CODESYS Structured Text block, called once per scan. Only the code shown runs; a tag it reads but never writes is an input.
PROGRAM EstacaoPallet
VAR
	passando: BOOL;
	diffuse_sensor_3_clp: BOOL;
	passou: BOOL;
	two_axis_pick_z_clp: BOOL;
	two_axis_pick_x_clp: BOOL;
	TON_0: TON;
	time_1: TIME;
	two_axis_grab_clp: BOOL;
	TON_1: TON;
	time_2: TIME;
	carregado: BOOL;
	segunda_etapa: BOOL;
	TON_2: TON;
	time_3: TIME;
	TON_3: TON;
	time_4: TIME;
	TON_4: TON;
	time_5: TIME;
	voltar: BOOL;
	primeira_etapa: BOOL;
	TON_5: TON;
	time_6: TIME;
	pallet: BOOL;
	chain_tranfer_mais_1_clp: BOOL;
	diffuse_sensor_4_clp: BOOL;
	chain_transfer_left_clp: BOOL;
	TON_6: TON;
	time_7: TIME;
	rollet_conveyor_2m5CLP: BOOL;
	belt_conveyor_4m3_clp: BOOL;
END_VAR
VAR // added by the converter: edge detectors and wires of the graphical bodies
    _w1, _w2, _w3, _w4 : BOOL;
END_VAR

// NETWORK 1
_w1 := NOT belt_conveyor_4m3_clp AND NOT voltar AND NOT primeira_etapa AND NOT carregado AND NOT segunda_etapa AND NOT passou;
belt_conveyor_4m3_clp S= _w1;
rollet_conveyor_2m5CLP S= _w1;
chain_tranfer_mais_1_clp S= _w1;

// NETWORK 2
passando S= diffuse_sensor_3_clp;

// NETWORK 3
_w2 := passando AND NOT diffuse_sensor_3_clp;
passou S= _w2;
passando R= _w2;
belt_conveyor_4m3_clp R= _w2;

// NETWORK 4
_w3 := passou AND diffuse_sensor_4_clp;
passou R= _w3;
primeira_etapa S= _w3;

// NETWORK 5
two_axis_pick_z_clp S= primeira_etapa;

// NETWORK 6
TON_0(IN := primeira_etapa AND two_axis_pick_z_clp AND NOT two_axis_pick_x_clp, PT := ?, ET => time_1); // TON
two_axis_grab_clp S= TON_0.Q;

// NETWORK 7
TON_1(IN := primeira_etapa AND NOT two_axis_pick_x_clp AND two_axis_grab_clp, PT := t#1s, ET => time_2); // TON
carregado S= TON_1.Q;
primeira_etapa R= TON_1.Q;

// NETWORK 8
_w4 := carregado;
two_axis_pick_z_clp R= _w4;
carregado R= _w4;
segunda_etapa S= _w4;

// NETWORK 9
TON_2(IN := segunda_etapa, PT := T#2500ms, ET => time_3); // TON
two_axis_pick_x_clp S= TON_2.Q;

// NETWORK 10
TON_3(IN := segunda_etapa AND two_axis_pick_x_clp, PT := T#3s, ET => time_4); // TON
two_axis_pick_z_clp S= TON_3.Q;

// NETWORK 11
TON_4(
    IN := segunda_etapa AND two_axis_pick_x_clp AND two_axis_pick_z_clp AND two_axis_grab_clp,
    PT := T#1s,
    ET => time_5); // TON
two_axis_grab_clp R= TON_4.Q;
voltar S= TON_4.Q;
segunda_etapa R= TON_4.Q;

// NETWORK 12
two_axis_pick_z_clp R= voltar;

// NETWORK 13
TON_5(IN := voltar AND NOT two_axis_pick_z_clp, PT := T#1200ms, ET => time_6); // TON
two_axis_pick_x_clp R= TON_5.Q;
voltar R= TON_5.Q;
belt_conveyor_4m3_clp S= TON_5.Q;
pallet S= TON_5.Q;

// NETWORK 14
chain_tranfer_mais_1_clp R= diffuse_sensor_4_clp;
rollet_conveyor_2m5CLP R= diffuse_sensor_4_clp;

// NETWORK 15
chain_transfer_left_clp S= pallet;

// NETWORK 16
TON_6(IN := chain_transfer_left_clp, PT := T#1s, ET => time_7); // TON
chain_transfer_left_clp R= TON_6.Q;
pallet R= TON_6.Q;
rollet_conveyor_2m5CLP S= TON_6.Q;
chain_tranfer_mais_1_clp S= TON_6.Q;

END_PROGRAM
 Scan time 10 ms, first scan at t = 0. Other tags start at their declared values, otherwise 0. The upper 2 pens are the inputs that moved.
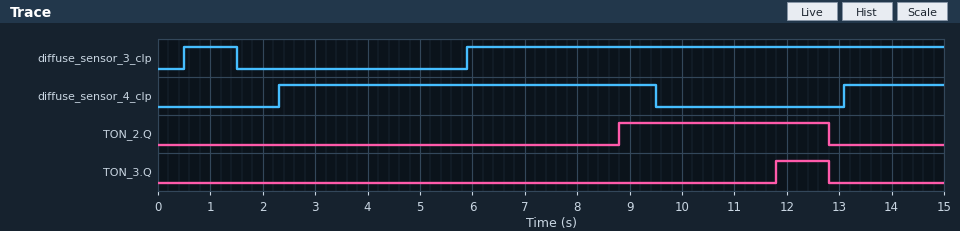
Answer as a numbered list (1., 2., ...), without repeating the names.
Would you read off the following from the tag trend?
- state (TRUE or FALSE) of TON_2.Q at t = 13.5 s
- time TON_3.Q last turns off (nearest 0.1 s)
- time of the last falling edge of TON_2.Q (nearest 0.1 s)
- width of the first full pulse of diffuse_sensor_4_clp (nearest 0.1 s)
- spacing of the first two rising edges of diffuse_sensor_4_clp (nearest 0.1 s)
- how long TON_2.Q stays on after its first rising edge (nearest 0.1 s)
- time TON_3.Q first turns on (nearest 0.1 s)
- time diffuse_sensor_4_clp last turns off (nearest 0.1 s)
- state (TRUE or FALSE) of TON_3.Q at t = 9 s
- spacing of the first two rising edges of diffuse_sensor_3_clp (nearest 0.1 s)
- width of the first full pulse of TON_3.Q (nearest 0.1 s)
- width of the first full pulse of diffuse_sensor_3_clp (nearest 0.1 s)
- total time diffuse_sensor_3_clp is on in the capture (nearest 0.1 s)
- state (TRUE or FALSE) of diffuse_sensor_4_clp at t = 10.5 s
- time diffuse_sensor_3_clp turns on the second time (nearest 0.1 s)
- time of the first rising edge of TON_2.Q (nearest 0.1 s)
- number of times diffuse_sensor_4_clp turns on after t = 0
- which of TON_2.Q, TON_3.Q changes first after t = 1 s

1. FALSE
2. 12.8 s
3. 12.8 s
4. 7.2 s
5. 10.8 s
6. 4.0 s
7. 11.8 s
8. 9.5 s
9. FALSE
10. 5.4 s
11. 1.0 s
12. 1.0 s
13. 10.1 s
14. FALSE
15. 5.9 s
16. 8.8 s
17. 2
18. TON_2.Q
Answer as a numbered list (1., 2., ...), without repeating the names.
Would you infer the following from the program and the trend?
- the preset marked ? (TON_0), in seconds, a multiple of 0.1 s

1. 3.0 s
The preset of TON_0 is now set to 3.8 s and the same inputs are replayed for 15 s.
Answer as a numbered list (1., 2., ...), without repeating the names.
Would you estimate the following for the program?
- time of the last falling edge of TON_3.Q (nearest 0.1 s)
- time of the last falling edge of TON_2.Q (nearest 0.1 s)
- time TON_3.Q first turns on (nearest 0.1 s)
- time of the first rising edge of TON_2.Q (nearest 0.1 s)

1. 13.6 s
2. 13.6 s
3. 12.6 s
4. 9.6 s
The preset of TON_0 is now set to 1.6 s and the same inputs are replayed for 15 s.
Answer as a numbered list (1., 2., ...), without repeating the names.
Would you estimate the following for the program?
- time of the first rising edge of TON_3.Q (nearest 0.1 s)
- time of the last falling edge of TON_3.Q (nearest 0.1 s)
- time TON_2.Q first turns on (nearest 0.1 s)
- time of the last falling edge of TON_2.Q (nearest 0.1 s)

1. 10.4 s
2. 11.4 s
3. 7.4 s
4. 11.4 s
